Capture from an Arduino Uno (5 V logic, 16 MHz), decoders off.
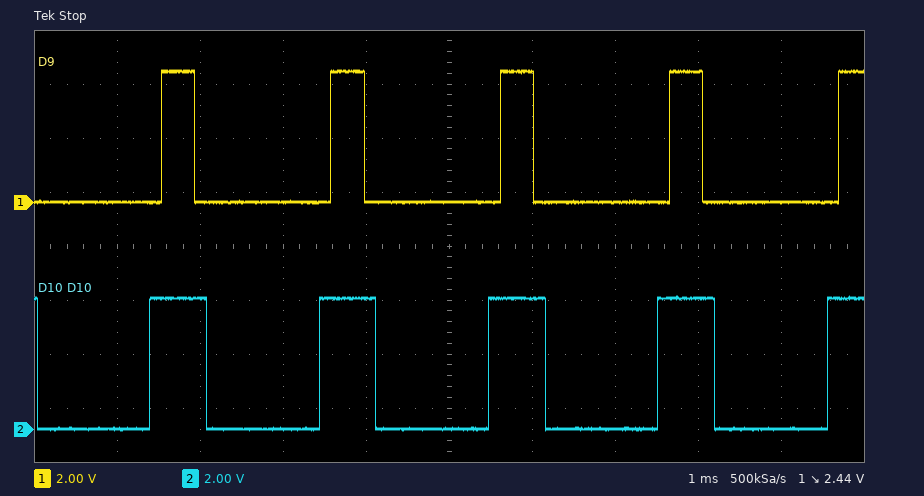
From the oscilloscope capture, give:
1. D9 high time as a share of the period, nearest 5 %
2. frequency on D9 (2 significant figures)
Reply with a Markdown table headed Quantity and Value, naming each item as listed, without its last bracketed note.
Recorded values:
| Quantity | Value |
|---|---|
| D9 high time as a share of the period, nearest 5 % | 20 % |
| frequency on D9 | 490 Hz |
